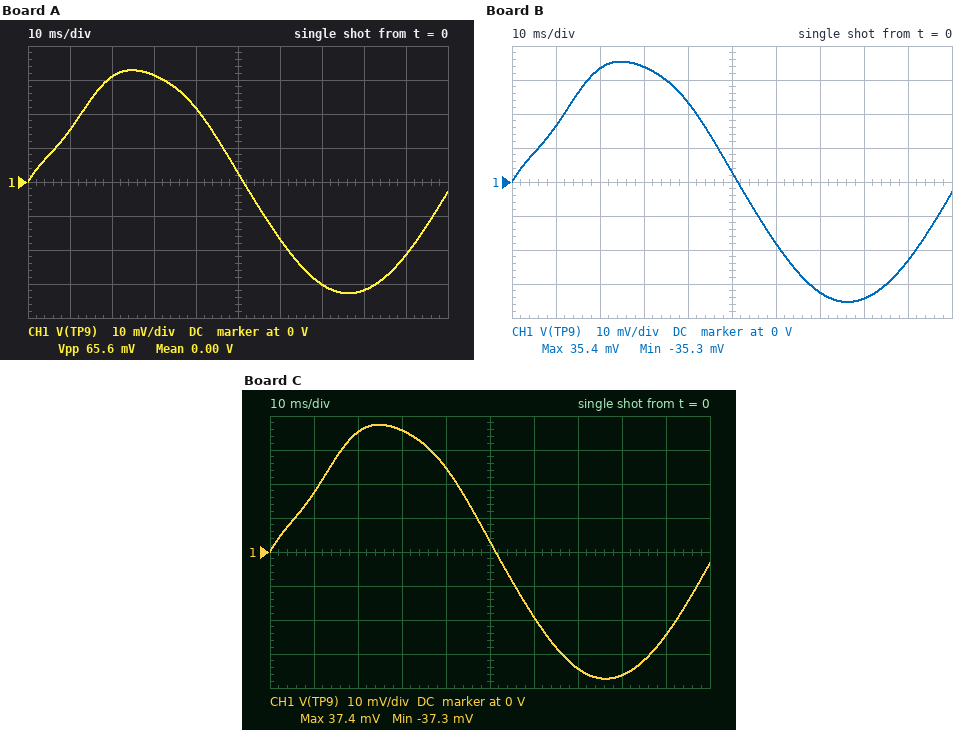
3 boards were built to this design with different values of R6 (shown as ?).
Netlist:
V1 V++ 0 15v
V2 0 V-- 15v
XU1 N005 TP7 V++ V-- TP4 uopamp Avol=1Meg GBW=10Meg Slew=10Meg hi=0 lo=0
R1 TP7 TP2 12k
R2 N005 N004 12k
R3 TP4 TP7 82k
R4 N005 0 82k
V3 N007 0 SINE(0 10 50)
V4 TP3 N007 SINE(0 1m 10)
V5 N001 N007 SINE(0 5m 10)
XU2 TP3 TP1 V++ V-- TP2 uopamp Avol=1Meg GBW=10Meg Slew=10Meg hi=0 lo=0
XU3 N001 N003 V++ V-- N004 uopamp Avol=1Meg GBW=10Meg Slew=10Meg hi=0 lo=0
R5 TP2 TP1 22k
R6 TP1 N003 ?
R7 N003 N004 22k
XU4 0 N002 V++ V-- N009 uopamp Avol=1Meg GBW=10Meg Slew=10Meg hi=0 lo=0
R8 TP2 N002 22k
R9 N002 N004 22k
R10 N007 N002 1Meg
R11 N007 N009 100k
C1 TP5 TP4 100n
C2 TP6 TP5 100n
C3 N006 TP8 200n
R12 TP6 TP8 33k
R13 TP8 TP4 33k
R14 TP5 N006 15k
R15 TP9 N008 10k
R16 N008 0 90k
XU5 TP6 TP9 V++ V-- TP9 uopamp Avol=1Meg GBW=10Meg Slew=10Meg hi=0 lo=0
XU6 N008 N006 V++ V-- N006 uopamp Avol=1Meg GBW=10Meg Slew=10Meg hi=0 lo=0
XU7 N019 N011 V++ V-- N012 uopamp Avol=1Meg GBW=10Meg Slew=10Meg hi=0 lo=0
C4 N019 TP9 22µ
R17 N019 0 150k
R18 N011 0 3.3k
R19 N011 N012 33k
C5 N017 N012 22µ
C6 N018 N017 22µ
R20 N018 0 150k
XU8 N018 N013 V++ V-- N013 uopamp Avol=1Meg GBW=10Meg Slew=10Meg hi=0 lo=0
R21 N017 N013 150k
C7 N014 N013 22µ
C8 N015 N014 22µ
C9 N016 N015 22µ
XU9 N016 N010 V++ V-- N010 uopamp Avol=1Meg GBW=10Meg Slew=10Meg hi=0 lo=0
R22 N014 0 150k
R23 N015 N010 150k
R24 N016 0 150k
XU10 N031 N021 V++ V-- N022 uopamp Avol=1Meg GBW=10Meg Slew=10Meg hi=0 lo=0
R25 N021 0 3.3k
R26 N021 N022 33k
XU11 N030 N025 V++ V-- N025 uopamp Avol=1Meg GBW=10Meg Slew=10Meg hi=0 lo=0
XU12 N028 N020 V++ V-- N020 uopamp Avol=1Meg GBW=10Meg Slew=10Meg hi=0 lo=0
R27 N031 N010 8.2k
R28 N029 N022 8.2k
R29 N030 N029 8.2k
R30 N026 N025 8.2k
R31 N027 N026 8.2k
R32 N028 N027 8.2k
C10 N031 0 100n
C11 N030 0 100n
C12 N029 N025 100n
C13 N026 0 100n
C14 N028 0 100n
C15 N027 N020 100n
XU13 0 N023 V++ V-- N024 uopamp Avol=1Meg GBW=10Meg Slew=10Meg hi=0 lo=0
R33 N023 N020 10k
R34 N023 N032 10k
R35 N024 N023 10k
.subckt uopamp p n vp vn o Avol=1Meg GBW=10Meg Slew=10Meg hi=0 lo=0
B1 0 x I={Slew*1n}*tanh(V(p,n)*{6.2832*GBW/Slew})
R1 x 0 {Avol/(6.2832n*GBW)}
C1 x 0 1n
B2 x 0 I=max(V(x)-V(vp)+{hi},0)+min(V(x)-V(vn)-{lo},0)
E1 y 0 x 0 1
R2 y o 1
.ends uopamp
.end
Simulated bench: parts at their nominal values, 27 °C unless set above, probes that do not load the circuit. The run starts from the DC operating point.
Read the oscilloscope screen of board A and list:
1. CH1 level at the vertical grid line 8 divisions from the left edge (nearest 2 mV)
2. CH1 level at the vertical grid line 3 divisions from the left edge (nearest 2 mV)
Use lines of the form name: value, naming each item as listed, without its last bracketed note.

CH1 level at the vertical grid line 8 divisions from the left edge: -32 mV
CH1 level at the vertical grid line 3 divisions from the left edge: 32 mV
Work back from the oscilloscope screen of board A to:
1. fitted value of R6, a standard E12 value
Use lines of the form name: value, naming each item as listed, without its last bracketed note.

fitted value of R6, a standard E12 value: 220 kΩ
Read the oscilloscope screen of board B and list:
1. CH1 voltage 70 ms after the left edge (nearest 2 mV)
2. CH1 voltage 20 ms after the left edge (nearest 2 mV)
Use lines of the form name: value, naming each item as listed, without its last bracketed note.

CH1 voltage 70 ms after the left edge: -32 mV
CH1 voltage 20 ms after the left edge: 34 mV
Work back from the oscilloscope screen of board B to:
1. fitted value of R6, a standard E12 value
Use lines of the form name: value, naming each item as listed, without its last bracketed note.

fitted value of R6, a standard E12 value: 150 kΩ
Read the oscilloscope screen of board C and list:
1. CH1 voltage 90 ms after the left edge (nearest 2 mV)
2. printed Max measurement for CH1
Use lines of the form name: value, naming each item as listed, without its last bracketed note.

CH1 voltage 90 ms after the left edge: -24 mV
printed Max measurement for CH1: 37.4 mV
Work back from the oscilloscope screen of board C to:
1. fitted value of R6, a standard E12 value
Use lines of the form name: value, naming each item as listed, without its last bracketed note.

fitted value of R6, a standard E12 value: 120 kΩ
